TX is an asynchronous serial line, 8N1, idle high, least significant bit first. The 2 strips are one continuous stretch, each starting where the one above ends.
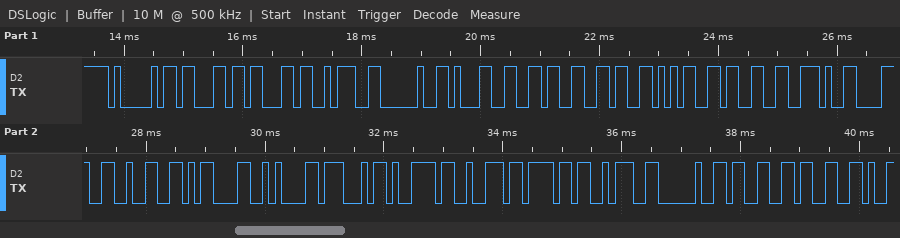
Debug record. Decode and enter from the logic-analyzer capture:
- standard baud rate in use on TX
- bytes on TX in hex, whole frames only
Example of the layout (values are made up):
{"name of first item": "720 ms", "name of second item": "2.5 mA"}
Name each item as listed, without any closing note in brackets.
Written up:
{"standard baud rate in use on TX": "9600 baud", "bytes on TX in hex, whole frames only": "41 63 63 3A 20 31 36 36 35 33 2E 38 32 0D 0A 47 79 72 6F 3A 20 33 33"}
